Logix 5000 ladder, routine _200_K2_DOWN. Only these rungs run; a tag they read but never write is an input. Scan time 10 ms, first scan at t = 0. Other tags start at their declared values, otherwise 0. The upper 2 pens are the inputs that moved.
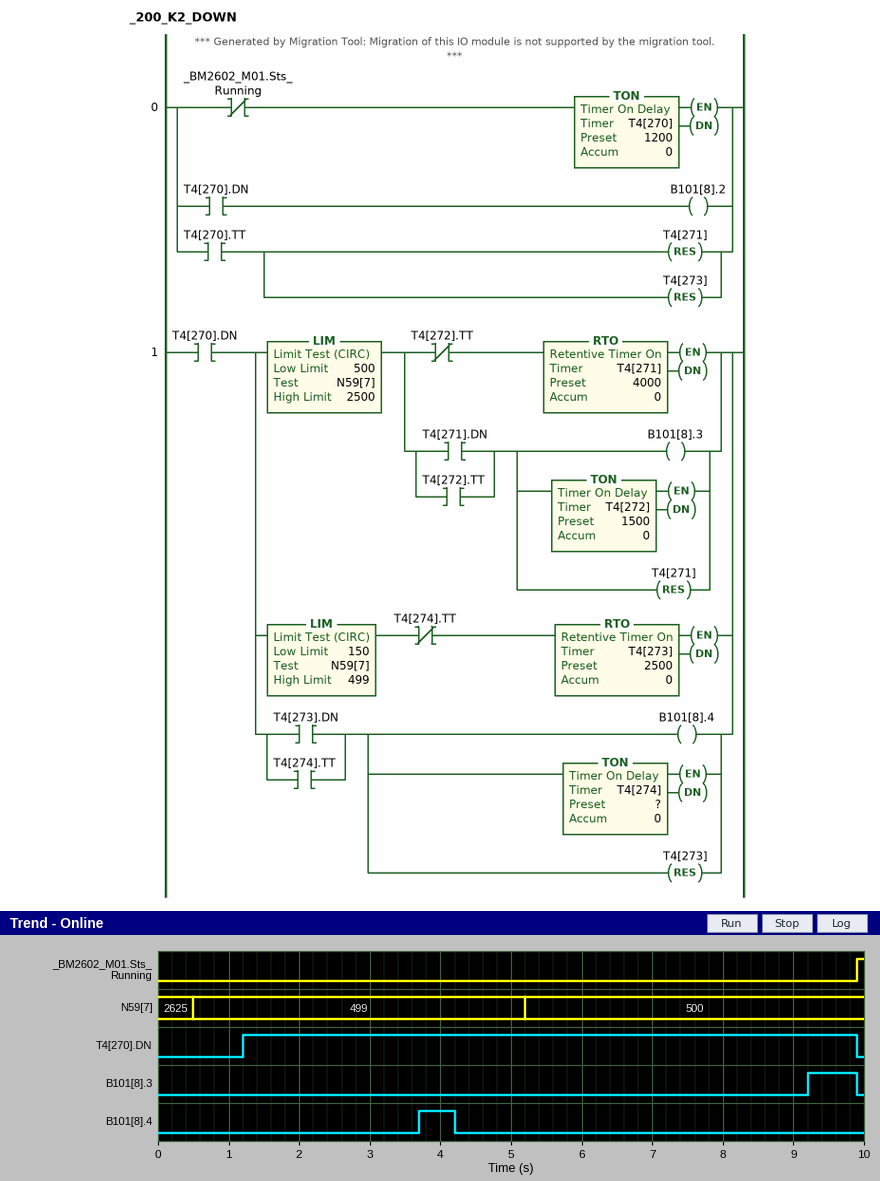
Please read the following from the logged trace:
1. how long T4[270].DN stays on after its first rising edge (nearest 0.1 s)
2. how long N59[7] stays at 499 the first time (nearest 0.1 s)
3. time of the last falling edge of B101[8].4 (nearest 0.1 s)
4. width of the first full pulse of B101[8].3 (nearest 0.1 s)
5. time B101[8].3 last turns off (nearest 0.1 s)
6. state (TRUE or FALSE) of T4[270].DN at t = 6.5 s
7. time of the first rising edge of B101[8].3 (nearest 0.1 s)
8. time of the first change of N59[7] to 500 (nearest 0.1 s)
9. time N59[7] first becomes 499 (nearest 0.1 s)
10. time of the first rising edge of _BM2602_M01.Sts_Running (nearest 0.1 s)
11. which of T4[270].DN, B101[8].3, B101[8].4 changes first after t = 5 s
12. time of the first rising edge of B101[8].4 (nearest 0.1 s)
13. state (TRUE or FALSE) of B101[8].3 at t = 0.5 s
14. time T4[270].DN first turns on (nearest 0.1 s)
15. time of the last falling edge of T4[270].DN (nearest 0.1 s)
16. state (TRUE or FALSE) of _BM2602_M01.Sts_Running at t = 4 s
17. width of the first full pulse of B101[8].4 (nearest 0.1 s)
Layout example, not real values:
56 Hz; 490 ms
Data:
8.7 s; 4.7 s; 4.2 s; 0.7 s; 9.9 s; TRUE; 9.2 s; 5.2 s; 0.5 s; 9.9 s; B101[8].3; 3.7 s; FALSE; 1.2 s; 9.9 s; FALSE; 0.5 s
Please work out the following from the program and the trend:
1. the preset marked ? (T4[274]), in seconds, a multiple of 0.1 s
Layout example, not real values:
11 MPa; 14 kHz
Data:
0.5 s
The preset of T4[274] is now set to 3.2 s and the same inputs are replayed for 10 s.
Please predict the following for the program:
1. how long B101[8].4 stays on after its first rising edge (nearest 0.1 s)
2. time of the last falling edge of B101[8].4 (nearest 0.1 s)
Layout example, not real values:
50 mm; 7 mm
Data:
3.2 s; 6.9 s
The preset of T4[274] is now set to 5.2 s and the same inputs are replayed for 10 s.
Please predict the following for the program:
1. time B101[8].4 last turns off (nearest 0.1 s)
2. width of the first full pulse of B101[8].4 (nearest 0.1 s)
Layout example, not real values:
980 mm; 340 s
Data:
8.9 s; 5.2 s
